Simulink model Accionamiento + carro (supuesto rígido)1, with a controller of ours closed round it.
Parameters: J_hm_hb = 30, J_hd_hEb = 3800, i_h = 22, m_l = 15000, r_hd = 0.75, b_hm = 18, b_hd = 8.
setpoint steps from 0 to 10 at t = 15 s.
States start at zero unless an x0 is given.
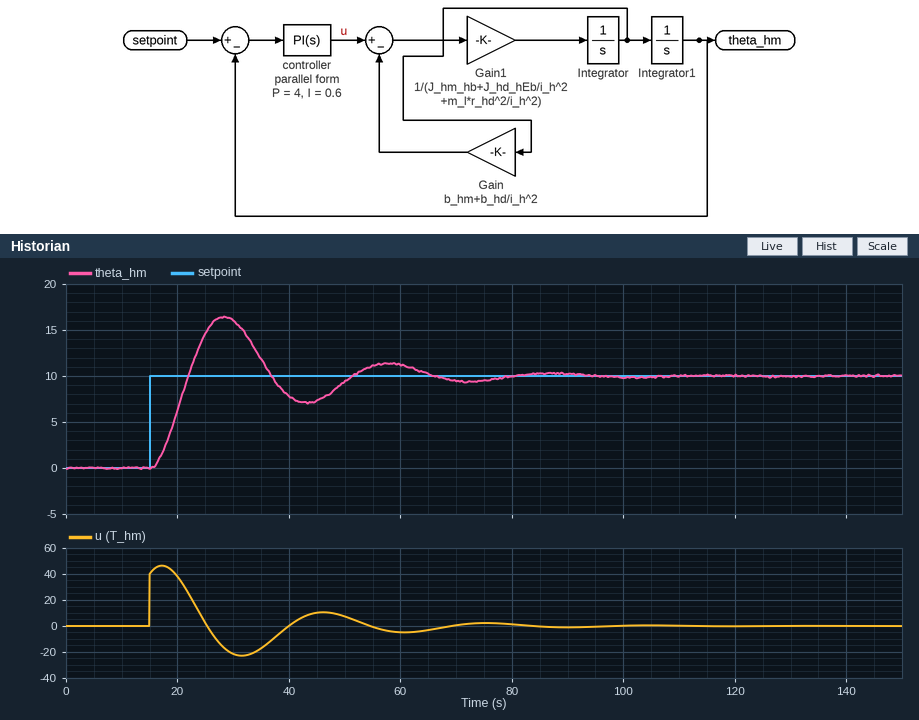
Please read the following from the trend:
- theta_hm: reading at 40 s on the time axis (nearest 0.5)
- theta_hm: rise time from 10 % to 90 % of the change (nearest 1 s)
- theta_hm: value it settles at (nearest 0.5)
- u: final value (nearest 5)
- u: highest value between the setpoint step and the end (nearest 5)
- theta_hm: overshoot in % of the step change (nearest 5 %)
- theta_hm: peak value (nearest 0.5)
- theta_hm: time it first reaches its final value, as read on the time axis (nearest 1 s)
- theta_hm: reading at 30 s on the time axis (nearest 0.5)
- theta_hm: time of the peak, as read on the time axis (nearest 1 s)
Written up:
8.0
5 s
10.0
0
45
65 %
16.5
22 s
16.0
28 s
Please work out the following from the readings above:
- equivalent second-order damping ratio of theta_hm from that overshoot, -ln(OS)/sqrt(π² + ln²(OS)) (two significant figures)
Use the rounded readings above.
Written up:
0.14
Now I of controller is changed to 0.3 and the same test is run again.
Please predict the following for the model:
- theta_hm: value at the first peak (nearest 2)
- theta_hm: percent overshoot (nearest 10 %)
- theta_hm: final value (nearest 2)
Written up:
14
40 %
10
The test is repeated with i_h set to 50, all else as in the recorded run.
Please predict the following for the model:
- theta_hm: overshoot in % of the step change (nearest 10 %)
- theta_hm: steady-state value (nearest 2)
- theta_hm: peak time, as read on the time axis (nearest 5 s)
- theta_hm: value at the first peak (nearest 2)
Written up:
50 %
10
25 s
14
